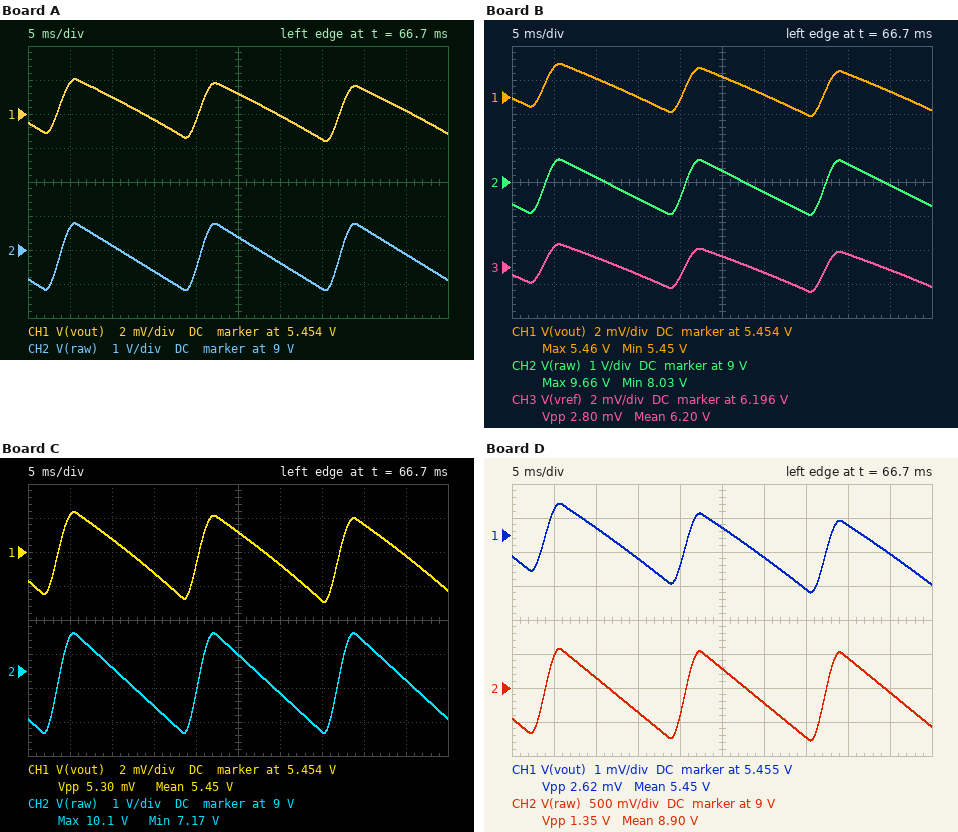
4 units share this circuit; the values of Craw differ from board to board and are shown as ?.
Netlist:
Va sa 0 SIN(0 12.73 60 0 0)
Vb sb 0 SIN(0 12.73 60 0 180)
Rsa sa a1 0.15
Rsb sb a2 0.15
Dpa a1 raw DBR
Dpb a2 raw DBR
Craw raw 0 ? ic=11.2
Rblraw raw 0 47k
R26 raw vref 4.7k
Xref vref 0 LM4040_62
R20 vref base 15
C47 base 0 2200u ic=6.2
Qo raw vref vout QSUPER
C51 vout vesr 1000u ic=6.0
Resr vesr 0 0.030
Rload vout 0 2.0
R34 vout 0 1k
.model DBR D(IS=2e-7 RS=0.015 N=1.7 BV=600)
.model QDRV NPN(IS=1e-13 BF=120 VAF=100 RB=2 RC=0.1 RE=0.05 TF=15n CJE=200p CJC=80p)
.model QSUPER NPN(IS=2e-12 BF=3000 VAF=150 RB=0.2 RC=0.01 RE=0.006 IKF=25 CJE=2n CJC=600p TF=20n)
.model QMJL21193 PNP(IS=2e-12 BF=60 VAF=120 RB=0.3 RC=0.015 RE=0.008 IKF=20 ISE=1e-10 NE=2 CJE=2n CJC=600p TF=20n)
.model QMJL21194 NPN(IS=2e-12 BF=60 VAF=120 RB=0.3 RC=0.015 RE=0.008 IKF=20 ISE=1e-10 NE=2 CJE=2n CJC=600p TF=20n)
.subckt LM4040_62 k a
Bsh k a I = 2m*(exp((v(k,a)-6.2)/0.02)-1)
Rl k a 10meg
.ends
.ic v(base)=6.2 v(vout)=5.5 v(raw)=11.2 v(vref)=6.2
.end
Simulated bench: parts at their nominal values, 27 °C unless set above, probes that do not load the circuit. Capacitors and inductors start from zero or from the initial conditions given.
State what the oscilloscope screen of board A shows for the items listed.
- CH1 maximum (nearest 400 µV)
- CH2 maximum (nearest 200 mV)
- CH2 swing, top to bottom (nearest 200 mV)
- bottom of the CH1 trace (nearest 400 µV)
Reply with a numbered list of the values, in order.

1. 5.4560 V
2. 9.8 V
3. 2.0 V
4. 5.4524 V
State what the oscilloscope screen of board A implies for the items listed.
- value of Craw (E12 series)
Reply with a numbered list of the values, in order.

1. 18 mF
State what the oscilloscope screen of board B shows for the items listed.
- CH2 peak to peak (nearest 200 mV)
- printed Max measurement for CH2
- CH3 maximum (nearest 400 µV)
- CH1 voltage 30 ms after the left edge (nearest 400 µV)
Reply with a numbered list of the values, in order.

1. 1.6 V
2. 9.66 V
3. 6.1972 V
4. 5.4540 V
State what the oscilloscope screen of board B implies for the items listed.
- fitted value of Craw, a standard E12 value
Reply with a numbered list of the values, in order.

1. 22 mF
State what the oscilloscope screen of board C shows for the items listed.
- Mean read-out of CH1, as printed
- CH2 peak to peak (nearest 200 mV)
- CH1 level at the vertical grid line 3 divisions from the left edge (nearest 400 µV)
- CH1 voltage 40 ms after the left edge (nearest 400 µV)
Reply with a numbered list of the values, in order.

1. 5.45 V
2. 3.0 V
3. 5.4528 V
4. 5.4556 V
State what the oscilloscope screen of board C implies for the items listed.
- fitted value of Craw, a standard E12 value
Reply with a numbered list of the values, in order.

1. 12 mF
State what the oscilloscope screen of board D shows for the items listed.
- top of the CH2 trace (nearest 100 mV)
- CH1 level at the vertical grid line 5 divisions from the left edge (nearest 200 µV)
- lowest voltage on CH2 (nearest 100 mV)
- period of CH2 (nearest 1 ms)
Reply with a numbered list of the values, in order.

1. 9.6 V
2. 5.4552 V
3. 8.2 V
4. 17 ms
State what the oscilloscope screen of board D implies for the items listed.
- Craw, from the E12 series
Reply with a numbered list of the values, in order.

1. 27 mF
